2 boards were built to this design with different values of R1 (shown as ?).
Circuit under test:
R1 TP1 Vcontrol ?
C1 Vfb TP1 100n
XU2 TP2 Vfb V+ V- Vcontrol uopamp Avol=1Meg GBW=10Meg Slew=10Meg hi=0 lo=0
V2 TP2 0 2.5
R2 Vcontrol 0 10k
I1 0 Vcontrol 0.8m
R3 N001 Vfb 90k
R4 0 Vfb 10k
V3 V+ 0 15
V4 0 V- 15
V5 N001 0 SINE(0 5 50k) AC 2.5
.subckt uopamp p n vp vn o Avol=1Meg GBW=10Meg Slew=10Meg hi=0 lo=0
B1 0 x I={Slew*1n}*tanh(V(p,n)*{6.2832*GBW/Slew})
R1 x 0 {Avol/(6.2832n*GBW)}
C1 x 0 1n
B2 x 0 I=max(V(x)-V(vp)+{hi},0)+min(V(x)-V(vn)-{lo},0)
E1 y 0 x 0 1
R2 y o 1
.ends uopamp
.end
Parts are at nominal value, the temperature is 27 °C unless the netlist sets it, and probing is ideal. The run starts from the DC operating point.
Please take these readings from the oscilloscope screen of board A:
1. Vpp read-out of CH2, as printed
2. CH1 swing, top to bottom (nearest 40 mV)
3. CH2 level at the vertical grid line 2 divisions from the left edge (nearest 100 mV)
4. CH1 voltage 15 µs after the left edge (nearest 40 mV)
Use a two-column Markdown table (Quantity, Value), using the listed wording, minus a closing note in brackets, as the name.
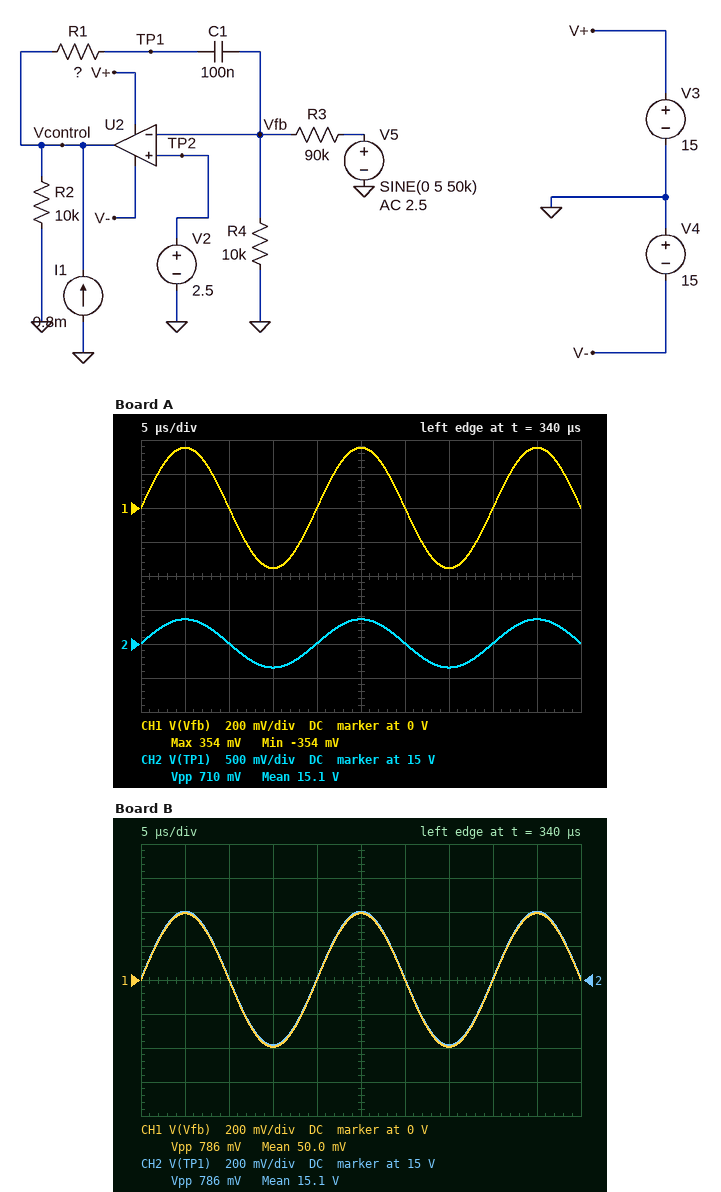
| Quantity | Value |
|---|---|
| Vpp read-out of CH2, as printed | 710 mV |
| CH1 swing, top to bottom | 720 mV |
| CH2 level at the vertical grid line 2 divisions from the left edge | 15.0 V |
| CH1 voltage 15 µs after the left edge | -360 mV |
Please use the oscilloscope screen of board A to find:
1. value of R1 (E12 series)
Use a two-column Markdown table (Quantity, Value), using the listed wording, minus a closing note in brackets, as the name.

| Quantity | Value |
|---|---|
| value of R1 | 22 kΩ |
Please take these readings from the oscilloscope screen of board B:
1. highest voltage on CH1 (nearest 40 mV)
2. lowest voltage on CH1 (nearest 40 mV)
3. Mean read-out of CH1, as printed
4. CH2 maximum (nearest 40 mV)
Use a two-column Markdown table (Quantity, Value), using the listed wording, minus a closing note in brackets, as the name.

| Quantity | Value |
|---|---|
| highest voltage on CH1 | 400 mV |
| lowest voltage on CH1 | -400 mV |
| Mean read-out of CH1, as printed | 50.0 mV |
| CH2 maximum | 15.40 V |
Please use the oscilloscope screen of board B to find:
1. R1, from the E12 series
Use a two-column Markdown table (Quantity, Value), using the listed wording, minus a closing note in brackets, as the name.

| Quantity | Value |
|---|---|
| R1, from the E12 series | 33 kΩ |
